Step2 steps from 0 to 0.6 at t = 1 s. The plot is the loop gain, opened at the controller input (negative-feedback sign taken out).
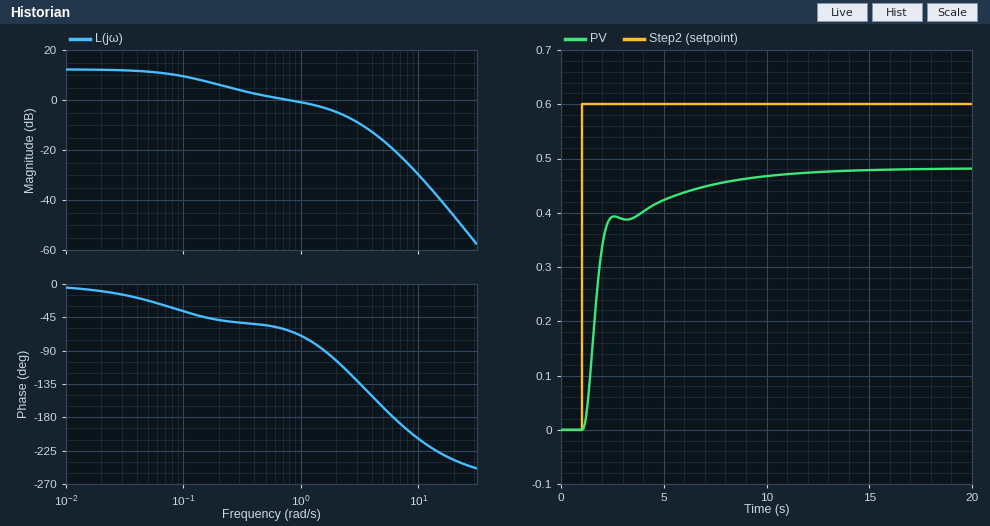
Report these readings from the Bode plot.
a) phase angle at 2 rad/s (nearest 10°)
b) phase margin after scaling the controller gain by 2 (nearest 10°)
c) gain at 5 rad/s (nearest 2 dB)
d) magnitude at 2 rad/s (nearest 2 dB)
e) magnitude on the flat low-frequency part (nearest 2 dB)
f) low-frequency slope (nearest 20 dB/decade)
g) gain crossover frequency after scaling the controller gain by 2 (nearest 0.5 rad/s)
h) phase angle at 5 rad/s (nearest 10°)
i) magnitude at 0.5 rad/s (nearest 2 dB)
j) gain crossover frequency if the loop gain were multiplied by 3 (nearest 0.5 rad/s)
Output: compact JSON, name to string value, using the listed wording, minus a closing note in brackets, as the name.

{"phase angle at 2 rad/s": "-100°", "phase margin after scaling the controller gain by 2": "70°", "gain at 5 rad/s": "-16 dB", "magnitude at 2 rad/s": "-4 dB", "magnitude on the flat low-frequency part": "12 dB", "low-frequency slope": "0 dB/decade", "gain crossover frequency after scaling the controller gain by 2": "2.5 rad/s", "phase angle at 5 rad/s": "-170°", "magnitude at 0.5 rad/s": "2 dB", "gain crossover frequency if the loop gain were multiplied by 3": "3.0 rad/s"}
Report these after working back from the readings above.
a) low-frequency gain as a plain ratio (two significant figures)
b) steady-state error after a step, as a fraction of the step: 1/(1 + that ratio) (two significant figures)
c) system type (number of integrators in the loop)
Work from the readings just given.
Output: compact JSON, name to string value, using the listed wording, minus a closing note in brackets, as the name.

{"low-frequency gain as a plain ratio": "4.0", "steady-state error after a step, as a fraction of the step: 1/(1 + that ratio)": "0.20", "system type": "0"}
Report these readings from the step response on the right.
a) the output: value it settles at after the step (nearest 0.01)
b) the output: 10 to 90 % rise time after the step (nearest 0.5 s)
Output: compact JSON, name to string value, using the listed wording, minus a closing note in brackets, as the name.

{"the output: value it settles at after the step": "0.48", "the output: 10 to 90 % rise time after the step": "4.5 s"}
